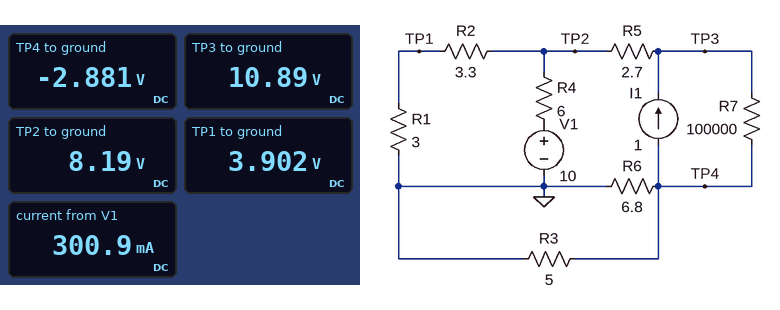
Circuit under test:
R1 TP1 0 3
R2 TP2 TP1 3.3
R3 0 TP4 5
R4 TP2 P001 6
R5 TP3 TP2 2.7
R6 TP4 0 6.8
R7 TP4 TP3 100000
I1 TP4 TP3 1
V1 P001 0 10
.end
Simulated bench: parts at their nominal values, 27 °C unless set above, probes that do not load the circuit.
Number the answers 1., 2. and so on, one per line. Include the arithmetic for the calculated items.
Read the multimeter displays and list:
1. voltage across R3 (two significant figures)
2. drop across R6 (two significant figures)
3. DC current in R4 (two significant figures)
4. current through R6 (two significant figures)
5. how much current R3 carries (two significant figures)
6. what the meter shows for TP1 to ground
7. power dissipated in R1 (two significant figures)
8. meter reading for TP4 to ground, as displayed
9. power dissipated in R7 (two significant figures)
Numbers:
1. 0 V - (-2.881 V) = 2.9 V
2. 0 V - (-2.881 V) = 2.9 V
3. (10 V - 8.19 V) / 6 Ω = 300 mA
4. (0 V - (-2.881 V)) / 6.8 Ω = 420 mA
5. (0 V - (-2.881 V)) / 5 Ω = 580 mA
6. 3.902 V
7. (3.902 V)^2 / 3 Ω = 5.1 W
8. -2.881 V
9. (10.89 V - (-2.881 V))^2 / 100 kΩ = 1.9 mW
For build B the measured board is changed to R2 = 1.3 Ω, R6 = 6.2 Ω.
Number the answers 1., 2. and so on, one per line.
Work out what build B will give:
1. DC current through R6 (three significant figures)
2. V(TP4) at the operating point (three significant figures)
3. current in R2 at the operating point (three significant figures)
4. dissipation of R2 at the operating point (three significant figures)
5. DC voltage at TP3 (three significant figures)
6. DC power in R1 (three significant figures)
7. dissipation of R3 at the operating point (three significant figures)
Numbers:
1. 446 mA
2. -2.77 V
3. 1.55 A
4. 3.14 W
5. 9.38 V
6. 7.24 W
7. 1.53 W
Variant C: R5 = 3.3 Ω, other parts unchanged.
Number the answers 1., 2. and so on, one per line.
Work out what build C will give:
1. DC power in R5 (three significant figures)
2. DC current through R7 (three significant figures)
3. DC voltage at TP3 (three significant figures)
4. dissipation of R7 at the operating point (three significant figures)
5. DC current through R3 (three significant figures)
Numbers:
1. 3.30 W
2. 144 µA
3. 11.5 V
4. 2.07 mW
5. 576 mA
